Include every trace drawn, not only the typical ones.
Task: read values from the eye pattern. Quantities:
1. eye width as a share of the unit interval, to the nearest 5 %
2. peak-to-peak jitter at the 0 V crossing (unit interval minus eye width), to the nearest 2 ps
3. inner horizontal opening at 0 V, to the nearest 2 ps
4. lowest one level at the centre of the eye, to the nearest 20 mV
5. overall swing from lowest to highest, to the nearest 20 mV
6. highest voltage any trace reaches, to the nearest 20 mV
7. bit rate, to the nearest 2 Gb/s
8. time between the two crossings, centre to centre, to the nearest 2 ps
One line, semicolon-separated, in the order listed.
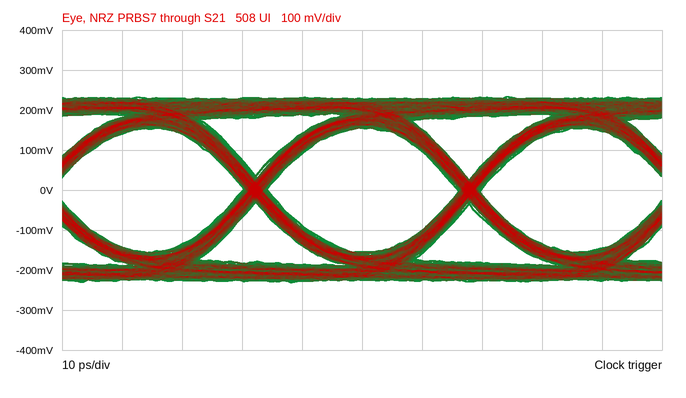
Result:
90 %; 4 ps; 32 ps; 160 mV; 460 mV; 240 mV; 28 Gb/s; 36 ps
